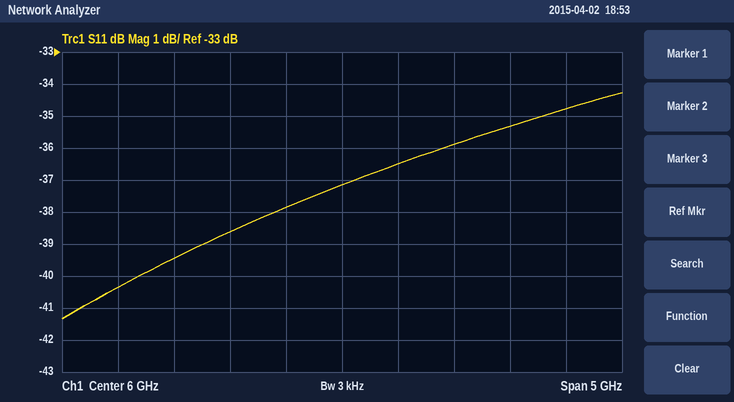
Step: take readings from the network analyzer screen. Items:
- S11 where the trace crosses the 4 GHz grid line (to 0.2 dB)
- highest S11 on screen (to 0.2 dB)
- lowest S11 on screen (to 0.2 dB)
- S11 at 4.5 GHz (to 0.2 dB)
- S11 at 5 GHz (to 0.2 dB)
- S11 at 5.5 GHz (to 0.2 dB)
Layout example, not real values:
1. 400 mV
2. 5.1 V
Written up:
1. -40.4 dB
2. -34.2 dB
3. -41.4 dB
4. -39.4 dB
5. -38.6 dB
6. -37.8 dB
